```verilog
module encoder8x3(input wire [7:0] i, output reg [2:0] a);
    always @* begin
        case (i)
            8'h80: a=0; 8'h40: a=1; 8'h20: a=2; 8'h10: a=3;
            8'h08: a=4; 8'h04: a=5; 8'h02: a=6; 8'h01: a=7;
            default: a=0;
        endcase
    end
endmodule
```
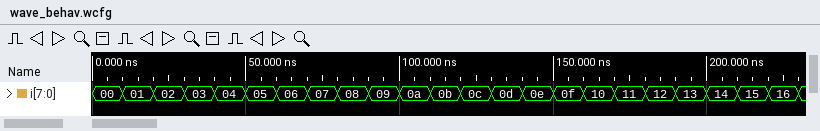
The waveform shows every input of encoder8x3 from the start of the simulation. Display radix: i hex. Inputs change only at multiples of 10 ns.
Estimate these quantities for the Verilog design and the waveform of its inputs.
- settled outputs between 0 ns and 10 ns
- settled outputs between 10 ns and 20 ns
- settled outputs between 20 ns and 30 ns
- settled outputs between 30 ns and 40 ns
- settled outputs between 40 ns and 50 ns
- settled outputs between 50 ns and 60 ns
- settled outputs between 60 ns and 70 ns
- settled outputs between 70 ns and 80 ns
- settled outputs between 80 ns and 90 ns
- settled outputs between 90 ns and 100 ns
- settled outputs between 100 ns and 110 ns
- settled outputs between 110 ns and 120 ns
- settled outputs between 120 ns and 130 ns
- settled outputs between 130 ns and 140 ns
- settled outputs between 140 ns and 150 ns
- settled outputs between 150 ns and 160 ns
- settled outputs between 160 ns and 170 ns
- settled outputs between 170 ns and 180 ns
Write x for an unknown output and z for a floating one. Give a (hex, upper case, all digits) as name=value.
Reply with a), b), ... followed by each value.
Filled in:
a) a=0
b) a=7
c) a=6
d) a=0
e) a=5
f) a=0
g) a=0
h) a=0
i) a=4
j) a=0
k) a=0
l) a=0
m) a=0
n) a=0
o) a=0
p) a=0
q) a=3
r) a=0
